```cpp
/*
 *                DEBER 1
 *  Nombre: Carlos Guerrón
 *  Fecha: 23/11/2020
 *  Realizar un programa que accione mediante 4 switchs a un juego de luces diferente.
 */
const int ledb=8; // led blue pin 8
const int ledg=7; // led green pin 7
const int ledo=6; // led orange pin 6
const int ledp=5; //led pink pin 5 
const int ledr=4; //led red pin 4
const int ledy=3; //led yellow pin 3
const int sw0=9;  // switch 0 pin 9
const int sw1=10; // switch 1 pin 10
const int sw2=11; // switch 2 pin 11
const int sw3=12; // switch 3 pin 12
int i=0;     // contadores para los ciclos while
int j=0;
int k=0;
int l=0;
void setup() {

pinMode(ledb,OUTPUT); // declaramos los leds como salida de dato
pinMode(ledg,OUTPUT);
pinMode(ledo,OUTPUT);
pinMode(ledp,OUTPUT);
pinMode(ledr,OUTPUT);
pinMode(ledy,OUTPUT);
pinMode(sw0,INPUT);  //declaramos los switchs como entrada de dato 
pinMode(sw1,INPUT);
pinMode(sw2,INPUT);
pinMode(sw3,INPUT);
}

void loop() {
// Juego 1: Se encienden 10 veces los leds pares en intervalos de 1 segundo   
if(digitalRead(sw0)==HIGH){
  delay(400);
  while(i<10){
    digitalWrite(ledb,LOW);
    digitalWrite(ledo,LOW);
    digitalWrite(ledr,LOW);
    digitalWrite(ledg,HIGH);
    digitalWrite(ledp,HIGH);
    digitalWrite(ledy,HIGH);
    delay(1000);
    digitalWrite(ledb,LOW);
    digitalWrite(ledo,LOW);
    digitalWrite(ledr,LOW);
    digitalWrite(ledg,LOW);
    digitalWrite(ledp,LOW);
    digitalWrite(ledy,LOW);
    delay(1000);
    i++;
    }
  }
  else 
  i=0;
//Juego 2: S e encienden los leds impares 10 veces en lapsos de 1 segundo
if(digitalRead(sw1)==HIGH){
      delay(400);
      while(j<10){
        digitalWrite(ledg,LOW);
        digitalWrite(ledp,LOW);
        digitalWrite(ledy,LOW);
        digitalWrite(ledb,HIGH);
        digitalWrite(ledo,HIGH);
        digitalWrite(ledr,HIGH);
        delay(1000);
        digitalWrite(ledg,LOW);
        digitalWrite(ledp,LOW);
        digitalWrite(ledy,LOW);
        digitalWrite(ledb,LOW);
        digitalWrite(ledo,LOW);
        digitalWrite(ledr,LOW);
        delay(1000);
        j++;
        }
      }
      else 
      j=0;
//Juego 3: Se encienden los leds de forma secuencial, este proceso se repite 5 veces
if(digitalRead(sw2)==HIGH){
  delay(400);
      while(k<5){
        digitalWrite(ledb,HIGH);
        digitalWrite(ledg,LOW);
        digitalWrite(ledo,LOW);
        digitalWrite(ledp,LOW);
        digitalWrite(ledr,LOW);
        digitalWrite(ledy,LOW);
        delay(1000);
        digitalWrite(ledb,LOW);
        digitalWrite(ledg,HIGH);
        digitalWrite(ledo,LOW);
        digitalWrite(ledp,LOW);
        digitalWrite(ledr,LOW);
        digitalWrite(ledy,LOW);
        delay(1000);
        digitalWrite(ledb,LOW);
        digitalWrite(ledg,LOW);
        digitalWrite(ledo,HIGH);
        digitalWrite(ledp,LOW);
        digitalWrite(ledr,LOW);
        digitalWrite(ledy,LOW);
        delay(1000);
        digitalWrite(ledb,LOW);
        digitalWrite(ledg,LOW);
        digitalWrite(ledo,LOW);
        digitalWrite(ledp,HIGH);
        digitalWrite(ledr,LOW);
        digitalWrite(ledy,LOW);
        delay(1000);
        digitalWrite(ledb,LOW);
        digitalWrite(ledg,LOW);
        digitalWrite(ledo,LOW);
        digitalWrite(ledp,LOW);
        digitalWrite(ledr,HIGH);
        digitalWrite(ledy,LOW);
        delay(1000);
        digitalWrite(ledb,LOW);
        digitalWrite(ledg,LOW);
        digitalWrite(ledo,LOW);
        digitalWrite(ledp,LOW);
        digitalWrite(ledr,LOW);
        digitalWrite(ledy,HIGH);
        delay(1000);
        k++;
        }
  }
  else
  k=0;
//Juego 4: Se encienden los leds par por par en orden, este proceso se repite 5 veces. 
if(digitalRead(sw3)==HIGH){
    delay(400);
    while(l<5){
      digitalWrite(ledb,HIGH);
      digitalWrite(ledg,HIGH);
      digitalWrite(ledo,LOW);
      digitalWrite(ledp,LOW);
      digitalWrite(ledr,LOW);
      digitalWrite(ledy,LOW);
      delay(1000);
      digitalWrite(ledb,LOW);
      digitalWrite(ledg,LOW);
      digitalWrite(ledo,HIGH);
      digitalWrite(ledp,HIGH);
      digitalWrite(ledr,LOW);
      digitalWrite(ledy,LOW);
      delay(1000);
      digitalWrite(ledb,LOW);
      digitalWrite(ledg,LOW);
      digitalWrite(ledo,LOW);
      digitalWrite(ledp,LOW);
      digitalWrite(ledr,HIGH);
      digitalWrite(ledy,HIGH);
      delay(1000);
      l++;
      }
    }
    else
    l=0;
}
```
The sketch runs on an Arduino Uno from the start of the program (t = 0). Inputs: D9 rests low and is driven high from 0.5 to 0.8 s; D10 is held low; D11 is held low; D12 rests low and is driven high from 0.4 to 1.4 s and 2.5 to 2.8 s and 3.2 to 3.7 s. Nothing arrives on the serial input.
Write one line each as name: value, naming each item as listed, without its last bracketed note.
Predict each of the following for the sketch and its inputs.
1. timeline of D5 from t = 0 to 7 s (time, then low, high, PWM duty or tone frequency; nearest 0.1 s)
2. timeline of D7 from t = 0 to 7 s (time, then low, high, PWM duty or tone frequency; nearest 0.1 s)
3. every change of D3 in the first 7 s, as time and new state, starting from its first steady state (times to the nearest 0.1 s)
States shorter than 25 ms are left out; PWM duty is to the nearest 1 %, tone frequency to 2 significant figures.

timeline of D5 from t = 0 to 7 s: 0 s low; 1.8 s high; 2.8 s low; 4.8 s high; 5.8 s low
timeline of D7 from t = 0 to 7 s: 0 s low; 0.8 s high; 1.8 s low; 3.8 s high; 4.8 s low; 6.8 s high
every change of D3 in the first 7 s, as time and new state, starting from its first steady state: 0 s low; 2.8 s high; 3.8 s low; 5.8 s high; 6.8 s low
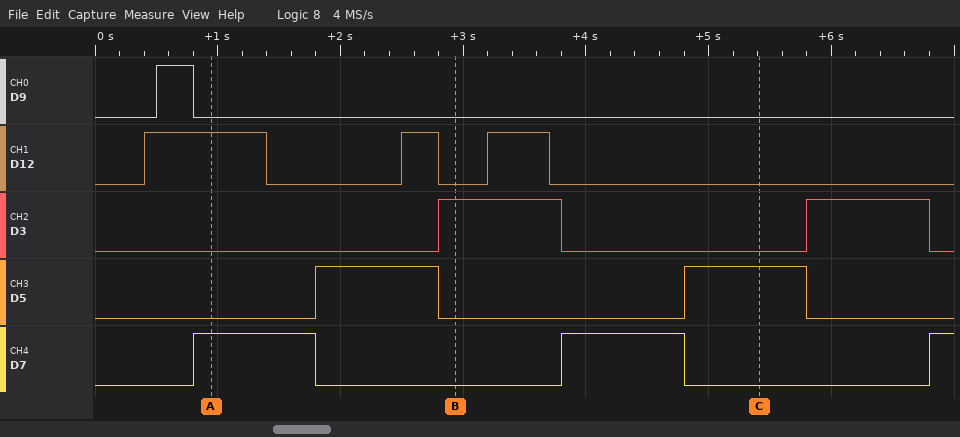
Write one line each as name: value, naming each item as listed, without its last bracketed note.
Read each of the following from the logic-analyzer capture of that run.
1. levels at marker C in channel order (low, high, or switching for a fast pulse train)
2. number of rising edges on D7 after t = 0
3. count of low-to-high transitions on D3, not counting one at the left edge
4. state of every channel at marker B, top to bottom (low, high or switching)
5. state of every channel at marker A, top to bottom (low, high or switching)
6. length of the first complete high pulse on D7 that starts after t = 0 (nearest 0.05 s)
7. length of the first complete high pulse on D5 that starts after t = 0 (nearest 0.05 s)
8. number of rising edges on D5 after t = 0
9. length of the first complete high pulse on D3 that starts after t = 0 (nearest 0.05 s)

levels at marker C in channel order: D9 low, D12 low, D3 low, D5 high, D7 low
number of rising edges on D7 after t = 0: 3
count of low-to-high transitions on D3, not counting one at the left edge: 2
state of every channel at marker B, top to bottom: D9 low, D12 low, D3 high, D5 low, D7 low
state of every channel at marker A, top to bottom: D9 low, D12 high, D3 low, D5 low, D7 high
length of the first complete high pulse on D7 that starts after t = 0: 1.00 s
length of the first complete high pulse on D5 that starts after t = 0: 1.00 s
number of rising edges on D5 after t = 0: 2
length of the first complete high pulse on D3 that starts after t = 0: 1.00 s
